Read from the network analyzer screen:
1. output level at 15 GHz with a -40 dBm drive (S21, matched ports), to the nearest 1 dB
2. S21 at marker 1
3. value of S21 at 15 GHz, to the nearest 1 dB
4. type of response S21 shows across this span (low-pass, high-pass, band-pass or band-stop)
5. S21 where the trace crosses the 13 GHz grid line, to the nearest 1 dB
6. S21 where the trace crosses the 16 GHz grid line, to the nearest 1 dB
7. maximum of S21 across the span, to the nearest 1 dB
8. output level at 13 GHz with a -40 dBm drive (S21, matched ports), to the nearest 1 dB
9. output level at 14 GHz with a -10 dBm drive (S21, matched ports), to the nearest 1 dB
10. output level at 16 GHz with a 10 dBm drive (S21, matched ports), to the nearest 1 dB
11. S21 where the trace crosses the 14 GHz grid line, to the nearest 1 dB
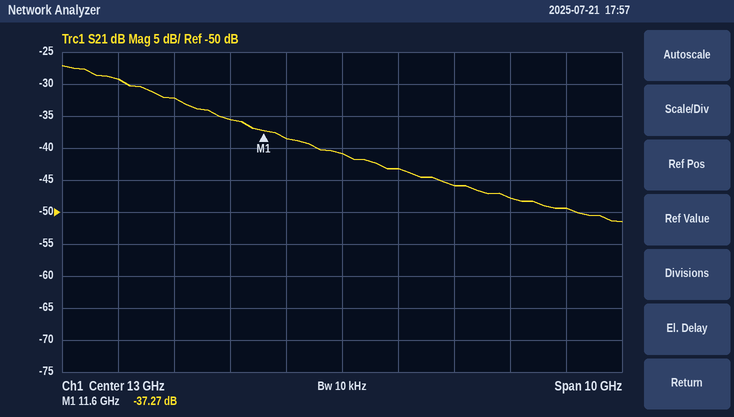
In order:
-86 dBm
-37.27 dB
-46 dB
low-pass
-41 dB
-48 dB
-27 dB
-81 dBm
-53 dBm
-38 dBm
-43 dB
